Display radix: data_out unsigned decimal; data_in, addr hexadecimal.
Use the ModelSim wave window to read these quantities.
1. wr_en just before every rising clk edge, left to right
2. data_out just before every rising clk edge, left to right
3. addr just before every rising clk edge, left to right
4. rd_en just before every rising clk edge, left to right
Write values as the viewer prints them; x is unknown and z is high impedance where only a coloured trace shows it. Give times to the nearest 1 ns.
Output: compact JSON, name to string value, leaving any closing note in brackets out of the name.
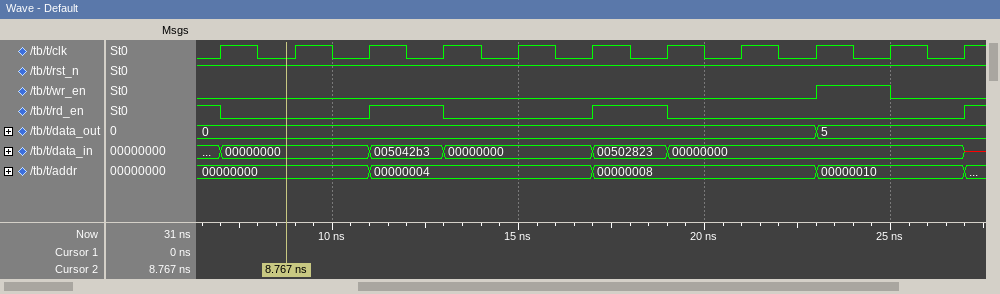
{"wr_en just before every rising clk edge, left to right": "0 0 0 0 0 0 0 0 0 1 0", "data_out just before every rising clk edge, left to right": "0, 0, 0, 0, 0, 0, 0, 0, 0, 5, 5", "addr just before every rising clk edge, left to right": "00000000, 00000000, 00000000, 00000004, 00000004, 00000004, 00000008, 00000008, 00000008, 00000010, 00000010", "rd_en just before every rising clk edge, left to right": "1 0 0 1 0 0 1 0 0 0 0"}
